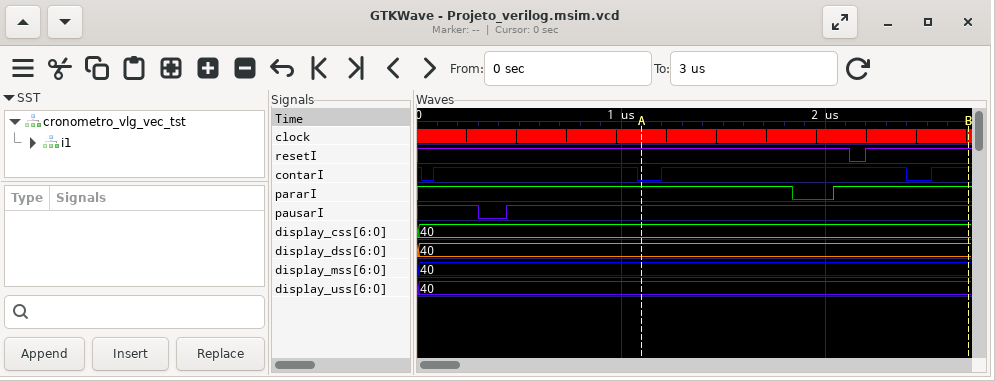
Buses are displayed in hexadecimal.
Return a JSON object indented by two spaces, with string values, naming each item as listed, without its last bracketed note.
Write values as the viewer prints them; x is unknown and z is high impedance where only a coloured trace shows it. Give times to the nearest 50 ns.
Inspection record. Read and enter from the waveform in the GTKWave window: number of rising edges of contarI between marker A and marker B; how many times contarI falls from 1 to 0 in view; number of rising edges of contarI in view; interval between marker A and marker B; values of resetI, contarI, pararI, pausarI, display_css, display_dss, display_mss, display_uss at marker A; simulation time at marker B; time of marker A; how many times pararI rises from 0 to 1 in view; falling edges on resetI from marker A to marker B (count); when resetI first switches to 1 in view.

{
  "number of rising edges of contarI between marker A and marker B": "2",
  "how many times contarI falls from 1 to 0 in view": "3",
  "number of rising edges of contarI in view": "3",
  "interval between marker A and marker B": "1600 ns",
  "values of resetI, contarI, pararI, pausarI, display_css, display_dss, display_mss, display_uss at marker A": "resetI=1, contarI=0, pararI=1, pausarI=1, display_css=40, display_dss=40, display_mss=40, display_uss=40",
  "simulation time at marker B": "2700 ns",
  "time of marker A": "1100 ns",
  "how many times pararI rises from 0 to 1 in view": "1",
  "falling edges on resetI from marker A to marker B": "1",
  "when resetI first switches to 1 in view": "2200 ns"
}
